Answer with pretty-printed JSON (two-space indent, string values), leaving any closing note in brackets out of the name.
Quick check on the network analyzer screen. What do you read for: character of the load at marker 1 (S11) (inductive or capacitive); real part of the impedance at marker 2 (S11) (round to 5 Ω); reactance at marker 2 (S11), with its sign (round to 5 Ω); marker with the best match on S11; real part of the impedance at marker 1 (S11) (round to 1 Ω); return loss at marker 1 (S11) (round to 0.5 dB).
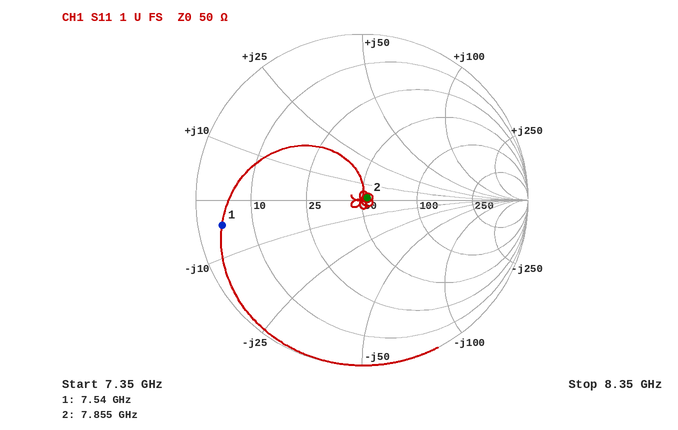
{
  "character of the load at marker 1 (S11)": "capacitive",
  "real part of the impedance at marker 2 (S11)": "55 Ω",
  "reactance at marker 2 (S11), with its sign": "0 Ω",
  "marker with the best match on S11": "marker 2",
  "real part of the impedance at marker 1 (S11)": "4 Ω",
  "return loss at marker 1 (S11)": "1.5 dB"
}
